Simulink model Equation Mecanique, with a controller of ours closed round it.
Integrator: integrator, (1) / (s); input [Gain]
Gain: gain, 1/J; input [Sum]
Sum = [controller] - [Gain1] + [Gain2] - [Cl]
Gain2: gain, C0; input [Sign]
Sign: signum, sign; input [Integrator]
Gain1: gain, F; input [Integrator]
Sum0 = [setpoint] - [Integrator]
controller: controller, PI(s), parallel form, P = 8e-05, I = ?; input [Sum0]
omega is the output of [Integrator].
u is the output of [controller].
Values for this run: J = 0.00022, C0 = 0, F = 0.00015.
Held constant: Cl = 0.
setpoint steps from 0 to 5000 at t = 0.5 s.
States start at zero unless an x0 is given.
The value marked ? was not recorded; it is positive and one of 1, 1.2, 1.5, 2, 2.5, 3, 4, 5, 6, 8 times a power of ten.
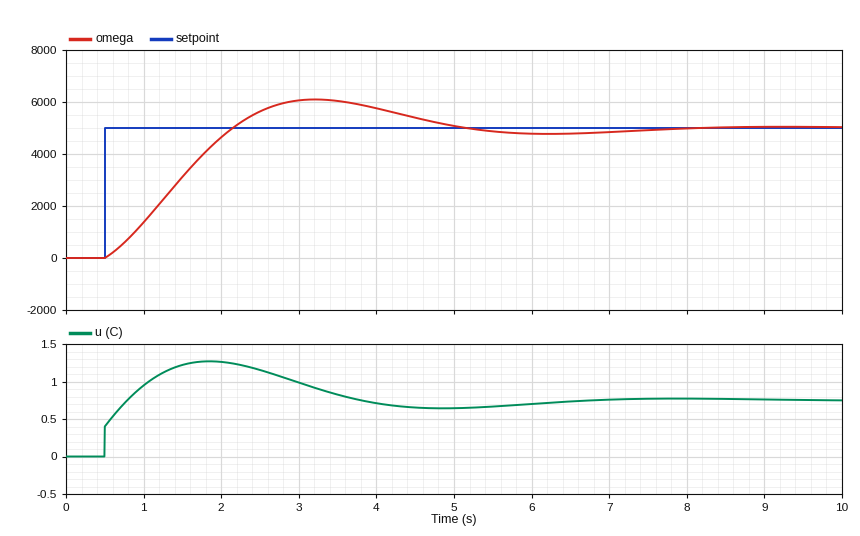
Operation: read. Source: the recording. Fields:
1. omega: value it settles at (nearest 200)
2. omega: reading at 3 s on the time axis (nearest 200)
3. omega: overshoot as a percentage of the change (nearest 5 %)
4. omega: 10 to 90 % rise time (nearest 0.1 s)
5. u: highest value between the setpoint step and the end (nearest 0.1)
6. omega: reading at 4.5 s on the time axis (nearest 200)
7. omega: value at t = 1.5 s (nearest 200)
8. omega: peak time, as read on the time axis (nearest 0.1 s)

5000
6000
20 %
1.2 s
1.3
5400
3200
3.2 s
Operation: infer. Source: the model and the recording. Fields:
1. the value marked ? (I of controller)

0.0003
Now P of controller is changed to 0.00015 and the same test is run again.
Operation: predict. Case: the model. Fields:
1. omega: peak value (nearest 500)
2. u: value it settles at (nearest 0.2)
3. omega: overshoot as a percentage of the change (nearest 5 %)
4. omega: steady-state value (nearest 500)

5500
0.8
15 %
5000
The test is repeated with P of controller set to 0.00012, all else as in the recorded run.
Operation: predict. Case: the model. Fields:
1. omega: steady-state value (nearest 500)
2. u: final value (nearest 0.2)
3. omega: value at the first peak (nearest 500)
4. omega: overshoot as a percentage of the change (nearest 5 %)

5000
0.8
6000
15 %
